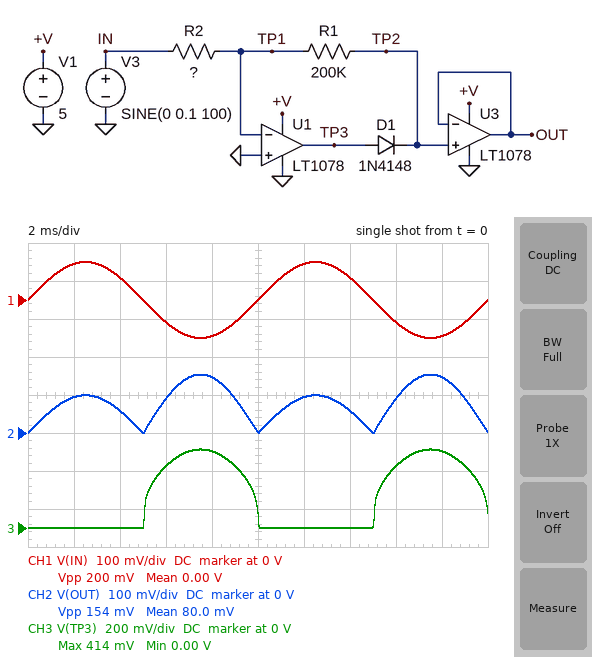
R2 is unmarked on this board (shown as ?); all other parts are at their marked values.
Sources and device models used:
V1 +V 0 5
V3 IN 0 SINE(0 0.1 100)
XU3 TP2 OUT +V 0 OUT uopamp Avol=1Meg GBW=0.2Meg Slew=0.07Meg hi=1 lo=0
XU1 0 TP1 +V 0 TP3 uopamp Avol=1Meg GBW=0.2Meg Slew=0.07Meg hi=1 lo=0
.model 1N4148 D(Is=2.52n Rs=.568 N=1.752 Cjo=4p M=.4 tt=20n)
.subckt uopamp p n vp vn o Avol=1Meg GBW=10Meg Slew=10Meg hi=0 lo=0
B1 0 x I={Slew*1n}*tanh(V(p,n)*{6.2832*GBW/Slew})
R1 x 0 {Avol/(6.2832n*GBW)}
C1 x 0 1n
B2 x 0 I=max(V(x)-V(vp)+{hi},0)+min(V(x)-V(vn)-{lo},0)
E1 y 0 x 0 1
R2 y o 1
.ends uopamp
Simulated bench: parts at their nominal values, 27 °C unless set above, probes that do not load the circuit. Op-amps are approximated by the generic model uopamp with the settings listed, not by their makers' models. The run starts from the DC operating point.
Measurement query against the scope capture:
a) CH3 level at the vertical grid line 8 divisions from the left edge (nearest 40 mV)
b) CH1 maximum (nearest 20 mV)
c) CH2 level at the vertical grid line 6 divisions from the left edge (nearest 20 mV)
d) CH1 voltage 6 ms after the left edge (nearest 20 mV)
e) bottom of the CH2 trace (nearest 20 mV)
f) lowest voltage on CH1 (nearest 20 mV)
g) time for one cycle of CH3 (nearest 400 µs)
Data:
320 mV
100 mV
100 mV
-60 mV
0 V
-100 mV
10.0 ms
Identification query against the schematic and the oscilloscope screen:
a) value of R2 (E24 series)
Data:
130 kΩ
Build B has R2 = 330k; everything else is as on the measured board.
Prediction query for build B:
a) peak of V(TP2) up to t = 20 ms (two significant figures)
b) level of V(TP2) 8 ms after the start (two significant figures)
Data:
99 mV
58 mV
